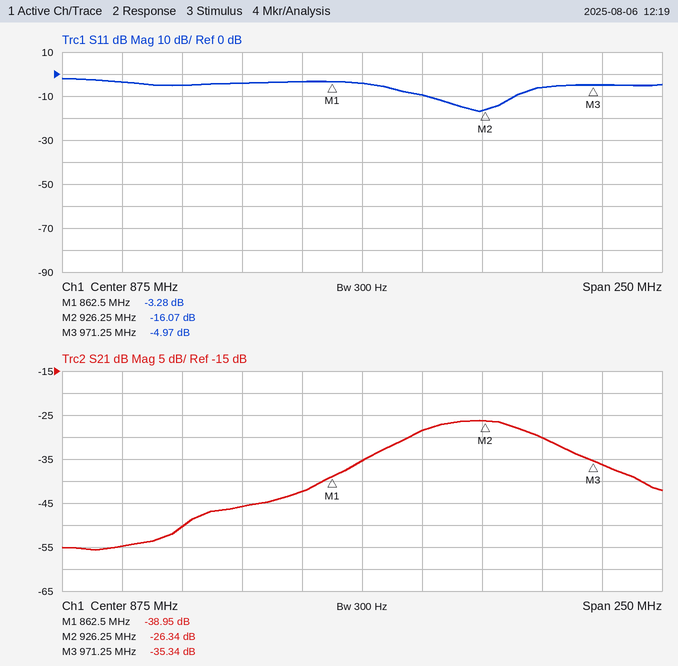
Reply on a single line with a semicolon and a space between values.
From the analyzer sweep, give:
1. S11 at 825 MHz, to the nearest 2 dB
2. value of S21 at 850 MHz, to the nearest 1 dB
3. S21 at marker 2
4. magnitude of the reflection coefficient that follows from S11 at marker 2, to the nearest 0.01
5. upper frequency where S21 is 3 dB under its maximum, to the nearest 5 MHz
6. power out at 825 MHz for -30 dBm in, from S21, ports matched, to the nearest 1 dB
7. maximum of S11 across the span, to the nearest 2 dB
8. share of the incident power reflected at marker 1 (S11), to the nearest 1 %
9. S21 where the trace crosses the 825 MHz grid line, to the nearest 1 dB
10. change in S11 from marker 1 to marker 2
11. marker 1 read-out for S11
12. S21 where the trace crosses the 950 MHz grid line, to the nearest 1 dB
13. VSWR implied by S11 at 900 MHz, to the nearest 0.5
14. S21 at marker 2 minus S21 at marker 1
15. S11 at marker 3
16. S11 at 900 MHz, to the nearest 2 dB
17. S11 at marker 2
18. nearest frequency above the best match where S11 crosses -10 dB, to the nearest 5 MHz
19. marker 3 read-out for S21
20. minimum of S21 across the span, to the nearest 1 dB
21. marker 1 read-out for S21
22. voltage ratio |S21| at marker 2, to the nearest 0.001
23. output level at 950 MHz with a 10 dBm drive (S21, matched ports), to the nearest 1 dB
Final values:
-4 dB; -42 dB; -26.34 dB; 0.16; 945 MHz; -76 dBm; -2 dB; 47 %; -46 dB; -12.79 dB; -3.28 dB; -30 dB; 2.0; 12.61 dB; -4.97 dB; -10 dB; -16.07 dB; 940 MHz; -35.34 dB; -56 dB; -38.95 dB; 0.048; -20 dBm
